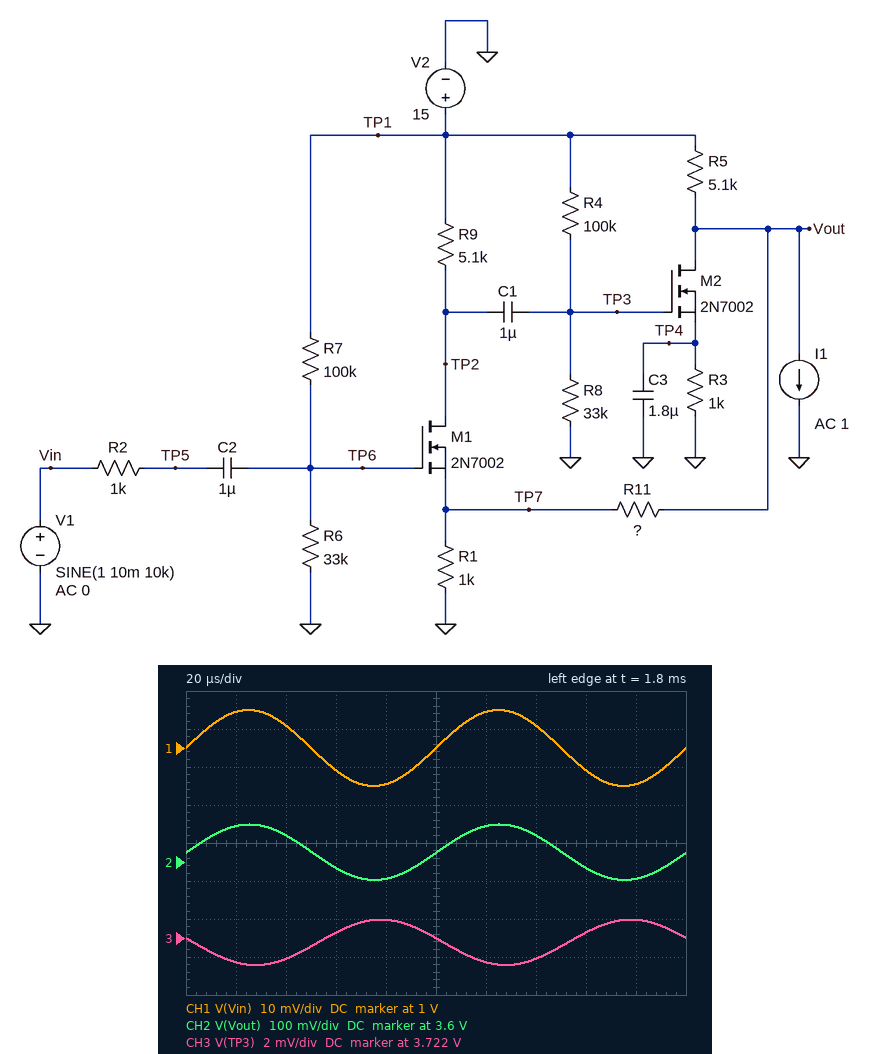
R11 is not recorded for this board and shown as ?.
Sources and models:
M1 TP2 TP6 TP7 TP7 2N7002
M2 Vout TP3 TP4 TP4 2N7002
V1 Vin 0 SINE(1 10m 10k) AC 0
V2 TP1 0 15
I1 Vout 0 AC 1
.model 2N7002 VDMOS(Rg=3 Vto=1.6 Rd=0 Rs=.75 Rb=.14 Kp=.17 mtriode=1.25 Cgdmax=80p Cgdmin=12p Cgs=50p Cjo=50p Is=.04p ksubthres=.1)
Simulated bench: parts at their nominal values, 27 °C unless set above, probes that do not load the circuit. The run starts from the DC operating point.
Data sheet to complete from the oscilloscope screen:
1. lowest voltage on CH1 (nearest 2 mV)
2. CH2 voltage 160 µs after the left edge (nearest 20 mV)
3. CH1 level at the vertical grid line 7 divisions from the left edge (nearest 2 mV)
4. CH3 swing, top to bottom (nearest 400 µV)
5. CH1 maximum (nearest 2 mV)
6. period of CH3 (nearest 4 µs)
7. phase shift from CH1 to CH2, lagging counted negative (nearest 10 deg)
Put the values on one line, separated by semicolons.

990 mV; 3.58 V; 1.006 V; 2.4 mV; 1.010 V; 100 µs; 0 deg
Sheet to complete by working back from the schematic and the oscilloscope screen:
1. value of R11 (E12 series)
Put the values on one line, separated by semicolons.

6.8 kΩ
